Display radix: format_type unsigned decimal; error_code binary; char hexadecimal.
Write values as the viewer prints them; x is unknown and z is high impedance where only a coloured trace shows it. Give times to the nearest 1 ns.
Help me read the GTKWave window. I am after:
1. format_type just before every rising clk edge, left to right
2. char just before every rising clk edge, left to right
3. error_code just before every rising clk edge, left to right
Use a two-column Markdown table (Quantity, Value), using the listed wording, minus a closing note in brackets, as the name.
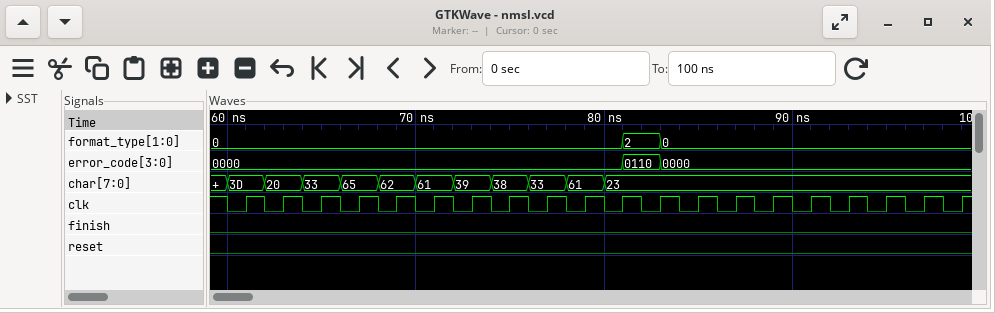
| Quantity | Value |
|---|---|
| format_type just before every rising clk edge, left to right | 0, 0, 0, 0, 0, 0, 0, 0, 0, 0, 0, 2, 0, 0, 0, 0, 0, 0, 0, 0 |
| char just before every rising clk edge, left to right | 3D, 20, 33, 65, 62, 61, 39, 38, 33, 61, 23, 23, 23, 23, 23, 23, 23, 23, 23, 23 |
| error_code just before every rising clk edge, left to right | 0000, 0000, 0000, 0000, 0000, 0000, 0000, 0000, 0000, 0000, 0000, 0110, 0000, 0000, 0000, 0000, 0000, 0000, 0000, 0000 |
